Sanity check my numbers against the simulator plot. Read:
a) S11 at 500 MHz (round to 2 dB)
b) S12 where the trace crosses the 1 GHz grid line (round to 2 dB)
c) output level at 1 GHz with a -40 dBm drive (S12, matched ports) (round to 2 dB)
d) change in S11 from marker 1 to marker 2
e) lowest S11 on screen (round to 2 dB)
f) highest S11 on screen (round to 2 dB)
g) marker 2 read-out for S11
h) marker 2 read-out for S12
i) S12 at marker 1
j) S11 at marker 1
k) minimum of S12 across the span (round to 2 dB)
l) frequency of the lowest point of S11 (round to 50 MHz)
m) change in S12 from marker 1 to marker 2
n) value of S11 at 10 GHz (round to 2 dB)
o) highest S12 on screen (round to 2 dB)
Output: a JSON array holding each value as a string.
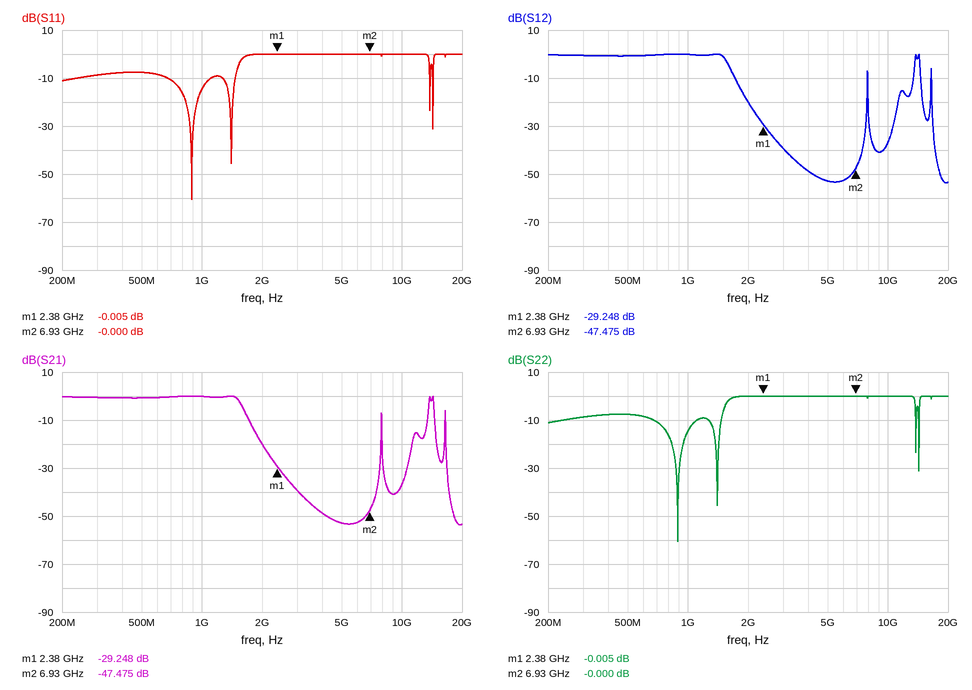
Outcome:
["-8 dB", "0 dB", "-40 dBm", "0.005 dB", "-60 dB", "0 dB", "-0.000 dB", "-47.475 dB", "-29.248 dB", "-0.005 dB", "-54 dB", "900 MHz", "-18.227 dB", "0 dB", "0 dB"]
